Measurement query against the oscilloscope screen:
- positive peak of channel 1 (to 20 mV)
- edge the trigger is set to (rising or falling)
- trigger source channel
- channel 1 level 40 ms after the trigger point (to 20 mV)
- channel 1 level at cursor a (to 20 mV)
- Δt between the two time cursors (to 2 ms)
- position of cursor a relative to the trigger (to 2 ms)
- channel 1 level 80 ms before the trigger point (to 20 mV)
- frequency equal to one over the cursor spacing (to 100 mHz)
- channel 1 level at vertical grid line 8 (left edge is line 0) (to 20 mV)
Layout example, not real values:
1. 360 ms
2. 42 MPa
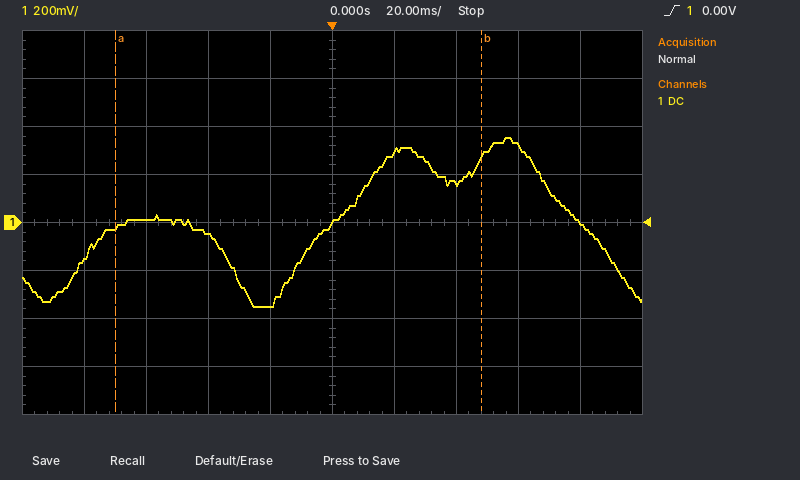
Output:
1. 360 mV
2. rising
3. channel 1
4. 160 mV
5. -20 mV
6. 118 ms
7. -70 ms
8. -160 mV
9. 8.5 Hz
10. 320 mV
